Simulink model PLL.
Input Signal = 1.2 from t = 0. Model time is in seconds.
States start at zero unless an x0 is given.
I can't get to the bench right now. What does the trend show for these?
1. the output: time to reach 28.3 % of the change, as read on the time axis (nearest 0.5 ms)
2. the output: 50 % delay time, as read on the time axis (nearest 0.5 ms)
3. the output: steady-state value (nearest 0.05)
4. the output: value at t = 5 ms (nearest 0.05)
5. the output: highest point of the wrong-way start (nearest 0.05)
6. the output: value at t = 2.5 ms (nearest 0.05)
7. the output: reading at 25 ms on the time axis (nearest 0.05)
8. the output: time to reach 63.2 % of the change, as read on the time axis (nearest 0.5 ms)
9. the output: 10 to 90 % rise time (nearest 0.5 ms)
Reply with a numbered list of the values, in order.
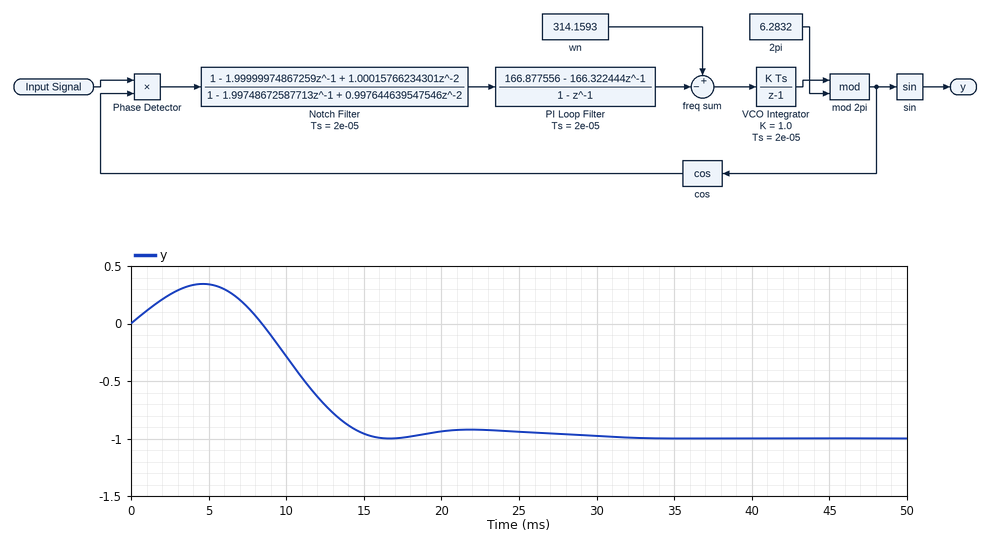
1. 10.0 ms
2. 11.0 ms
3. -1.00
4. 0.35
5. 0.35
6. 0.25
7. -0.95
8. 12.0 ms
9. 5.0 ms
